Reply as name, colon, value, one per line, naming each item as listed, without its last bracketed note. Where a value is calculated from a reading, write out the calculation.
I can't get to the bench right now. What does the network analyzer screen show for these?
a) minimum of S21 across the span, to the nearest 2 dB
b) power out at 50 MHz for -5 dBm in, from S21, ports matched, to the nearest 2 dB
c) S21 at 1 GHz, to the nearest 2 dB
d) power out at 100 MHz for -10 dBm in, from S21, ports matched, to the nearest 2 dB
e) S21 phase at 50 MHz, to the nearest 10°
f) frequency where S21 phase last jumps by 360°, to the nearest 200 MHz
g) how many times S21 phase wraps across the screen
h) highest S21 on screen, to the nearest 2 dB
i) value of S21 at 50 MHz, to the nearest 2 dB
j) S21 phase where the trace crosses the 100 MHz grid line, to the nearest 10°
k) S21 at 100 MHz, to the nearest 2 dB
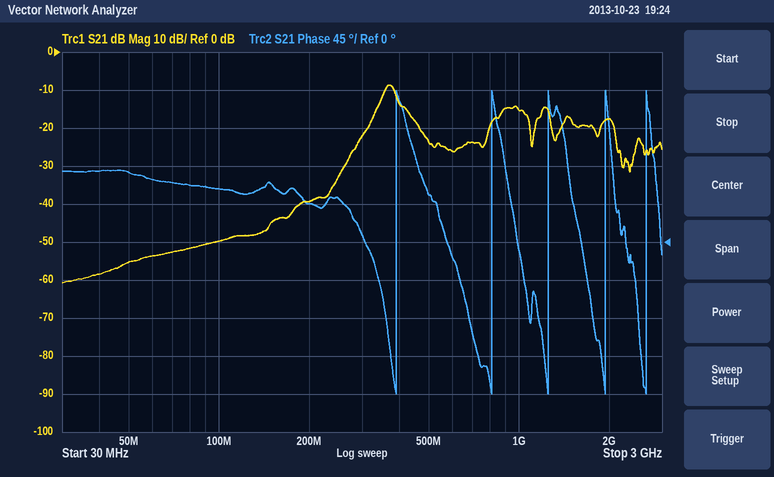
minimum of S21 across the span, to the nearest 2 dB: -60 dB
power out at 50 MHz for -5 dBm in, from S21, ports matched, to the nearest 2 dB: -5 dBm + (-56 dB) = -60 dBm
S21 at 1 GHz, to the nearest 2 dB: -16 dB
power out at 100 MHz for -10 dBm in, from S21, ports matched, to the nearest 2 dB: -10 dBm + (-50 dB) = -60 dBm
S21 phase at 50 MHz, to the nearest 10°: 80°
frequency where S21 phase last jumps by 360°, to the nearest 200 MHz: 2.6 GHz
how many times S21 phase wraps across the screen: 5
highest S21 on screen, to the nearest 2 dB: -8 dB
value of S21 at 50 MHz, to the nearest 2 dB: -56 dB
S21 phase where the trace crosses the 100 MHz grid line, to the nearest 10°: 60°
S21 at 100 MHz, to the nearest 2 dB: -50 dB
